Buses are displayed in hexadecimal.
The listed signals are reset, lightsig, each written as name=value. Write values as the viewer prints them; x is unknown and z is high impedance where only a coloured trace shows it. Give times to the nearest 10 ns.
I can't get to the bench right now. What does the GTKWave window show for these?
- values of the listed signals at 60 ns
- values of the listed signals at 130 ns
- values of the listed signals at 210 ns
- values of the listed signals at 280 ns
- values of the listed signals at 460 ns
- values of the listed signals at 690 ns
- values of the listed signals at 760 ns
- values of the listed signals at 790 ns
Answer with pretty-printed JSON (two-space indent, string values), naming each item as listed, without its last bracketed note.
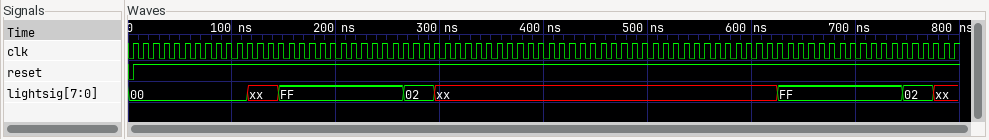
{
  "values of the listed signals at 60 ns": "reset=1, lightsig=00",
  "values of the listed signals at 130 ns": "reset=1, lightsig=xx",
  "values of the listed signals at 210 ns": "reset=1, lightsig=FF",
  "values of the listed signals at 280 ns": "reset=1, lightsig=02",
  "values of the listed signals at 460 ns": "reset=1, lightsig=xx",
  "values of the listed signals at 690 ns": "reset=1, lightsig=FF",
  "values of the listed signals at 760 ns": "reset=1, lightsig=02",
  "values of the listed signals at 790 ns": "reset=1, lightsig=xx"
}
